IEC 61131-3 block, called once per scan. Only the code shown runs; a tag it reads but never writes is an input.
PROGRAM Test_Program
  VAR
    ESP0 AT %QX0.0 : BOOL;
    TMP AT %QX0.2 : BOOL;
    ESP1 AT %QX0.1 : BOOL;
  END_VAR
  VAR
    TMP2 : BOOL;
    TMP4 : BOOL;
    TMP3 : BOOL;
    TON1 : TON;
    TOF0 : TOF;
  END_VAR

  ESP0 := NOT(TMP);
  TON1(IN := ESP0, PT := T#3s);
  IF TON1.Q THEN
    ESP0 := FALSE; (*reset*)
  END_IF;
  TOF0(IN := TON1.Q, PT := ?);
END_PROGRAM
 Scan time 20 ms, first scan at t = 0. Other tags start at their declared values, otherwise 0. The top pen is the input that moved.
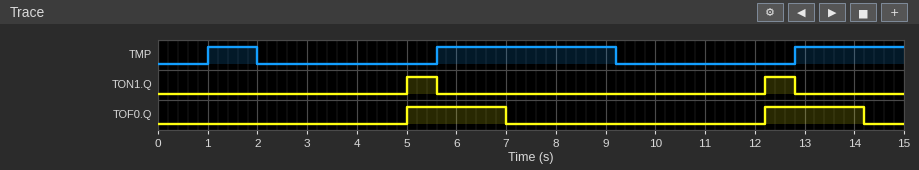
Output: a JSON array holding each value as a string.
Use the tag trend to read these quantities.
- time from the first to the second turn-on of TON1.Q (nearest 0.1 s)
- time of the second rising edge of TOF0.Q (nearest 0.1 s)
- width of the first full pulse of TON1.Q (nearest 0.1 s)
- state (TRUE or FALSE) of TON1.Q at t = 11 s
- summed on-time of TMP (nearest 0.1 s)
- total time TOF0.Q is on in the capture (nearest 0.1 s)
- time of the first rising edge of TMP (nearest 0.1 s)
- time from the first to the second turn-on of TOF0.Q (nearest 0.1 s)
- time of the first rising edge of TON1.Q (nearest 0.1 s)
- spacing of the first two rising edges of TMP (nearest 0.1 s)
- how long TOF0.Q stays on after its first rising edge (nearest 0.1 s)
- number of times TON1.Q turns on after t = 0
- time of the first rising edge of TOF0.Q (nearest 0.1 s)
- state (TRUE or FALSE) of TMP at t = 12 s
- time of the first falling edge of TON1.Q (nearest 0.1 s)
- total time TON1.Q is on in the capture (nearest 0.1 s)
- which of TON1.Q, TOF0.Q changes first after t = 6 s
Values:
["7.2 s", "12.2 s", "0.6 s", "FALSE", "6.8 s", "4.0 s", "1.0 s", "7.2 s", "5.0 s", "4.6 s", "2.0 s", "2", "5.0 s", "FALSE", "5.6 s", "1.2 s", "TOF0.Q"]
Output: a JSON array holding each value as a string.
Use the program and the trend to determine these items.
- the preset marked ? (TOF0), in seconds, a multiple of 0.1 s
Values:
["1.4 s"]
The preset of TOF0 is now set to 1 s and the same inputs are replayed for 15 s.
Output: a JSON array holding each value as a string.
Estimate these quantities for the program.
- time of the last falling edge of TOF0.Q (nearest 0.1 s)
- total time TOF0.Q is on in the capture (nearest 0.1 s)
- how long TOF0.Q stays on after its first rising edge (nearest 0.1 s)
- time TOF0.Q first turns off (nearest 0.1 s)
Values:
["13.8 s", "3.2 s", "1.6 s", "6.6 s"]
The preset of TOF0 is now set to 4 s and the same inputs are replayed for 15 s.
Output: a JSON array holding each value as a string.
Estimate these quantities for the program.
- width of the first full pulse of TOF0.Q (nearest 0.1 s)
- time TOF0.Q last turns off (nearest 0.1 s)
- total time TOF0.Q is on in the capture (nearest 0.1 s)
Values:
["4.6 s", "9.6 s", "7.4 s"]
